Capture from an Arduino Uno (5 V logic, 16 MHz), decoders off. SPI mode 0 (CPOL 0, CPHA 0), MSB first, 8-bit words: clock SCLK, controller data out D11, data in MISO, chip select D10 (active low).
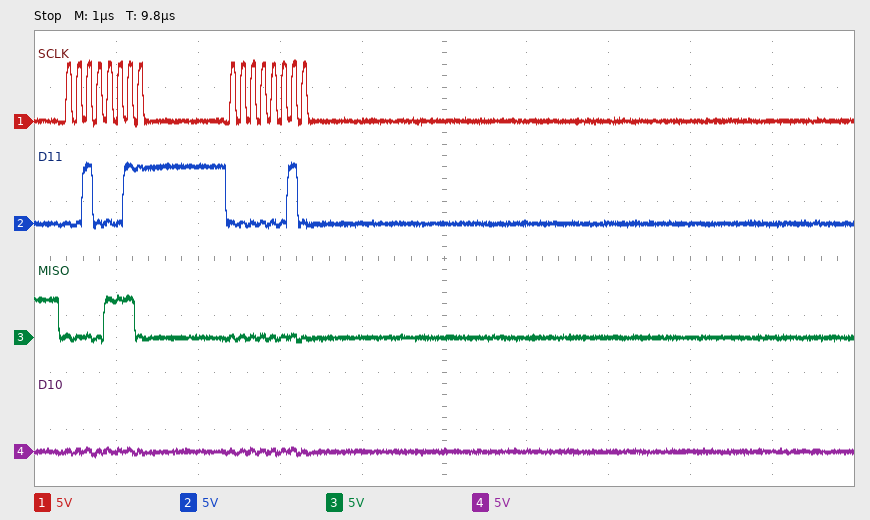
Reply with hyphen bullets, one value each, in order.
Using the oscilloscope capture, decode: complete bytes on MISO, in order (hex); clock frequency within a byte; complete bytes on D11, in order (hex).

- 0x0E 0x00
- 8 MHz
- 0x23 0x02
